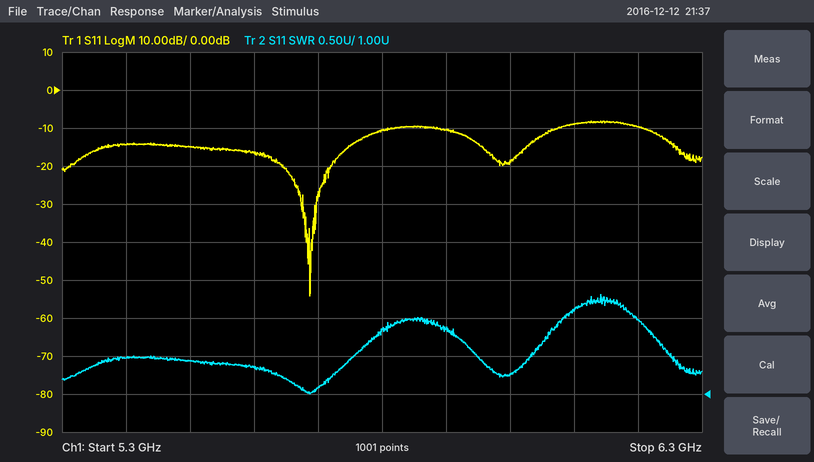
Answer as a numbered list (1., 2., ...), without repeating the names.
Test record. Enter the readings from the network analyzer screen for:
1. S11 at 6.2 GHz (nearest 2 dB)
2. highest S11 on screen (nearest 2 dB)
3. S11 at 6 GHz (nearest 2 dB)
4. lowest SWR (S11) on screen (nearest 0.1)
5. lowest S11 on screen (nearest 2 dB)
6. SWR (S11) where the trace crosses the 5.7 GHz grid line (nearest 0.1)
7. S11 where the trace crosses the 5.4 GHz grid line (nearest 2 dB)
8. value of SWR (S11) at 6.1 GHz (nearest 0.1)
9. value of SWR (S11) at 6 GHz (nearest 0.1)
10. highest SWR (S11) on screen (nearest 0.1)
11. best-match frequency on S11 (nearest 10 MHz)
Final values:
1. -10 dB
2. -8 dB
3. -18 dB
4. 1.0
5. -54 dB
6. 1.1
7. -14 dB
8. 2.1
9. 1.3
10. 2.3
11. 5.69 GHz
